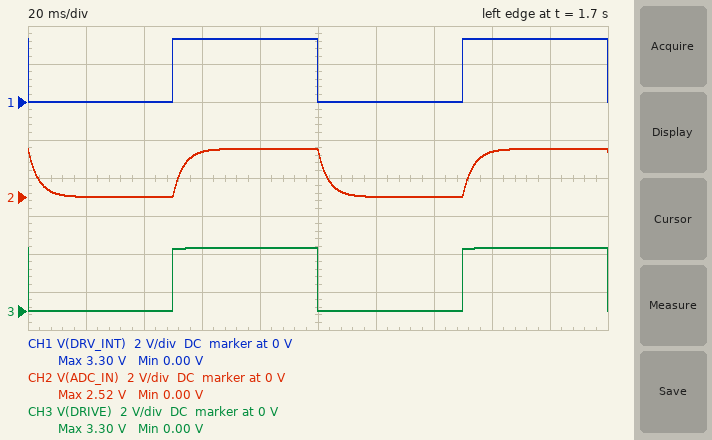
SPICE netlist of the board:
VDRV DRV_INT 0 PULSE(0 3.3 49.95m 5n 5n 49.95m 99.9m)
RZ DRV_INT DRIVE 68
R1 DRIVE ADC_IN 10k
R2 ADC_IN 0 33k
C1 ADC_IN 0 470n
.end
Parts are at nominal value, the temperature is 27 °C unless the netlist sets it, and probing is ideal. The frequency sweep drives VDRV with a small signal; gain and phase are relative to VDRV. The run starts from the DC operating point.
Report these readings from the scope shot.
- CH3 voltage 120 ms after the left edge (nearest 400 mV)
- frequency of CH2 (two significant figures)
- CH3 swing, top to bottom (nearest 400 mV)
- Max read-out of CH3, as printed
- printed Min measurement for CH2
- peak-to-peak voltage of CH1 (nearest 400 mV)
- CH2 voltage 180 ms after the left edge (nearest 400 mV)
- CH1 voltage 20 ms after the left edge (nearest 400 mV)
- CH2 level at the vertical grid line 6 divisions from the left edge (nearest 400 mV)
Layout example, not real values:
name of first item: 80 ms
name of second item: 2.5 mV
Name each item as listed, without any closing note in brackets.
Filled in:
CH3 voltage 120 ms after the left edge: 0 V
frequency of CH2: 10 Hz
CH3 swing, top to bottom: 3.2 V
Max read-out of CH3, as printed: 3.30 V
printed Min measurement for CH2: 0.00 V
peak-to-peak voltage of CH1: 3.2 V
CH2 voltage 180 ms after the left edge: 2.4 V
CH1 voltage 20 ms after the left edge: 0 V
CH2 level at the vertical grid line 6 divisions from the left edge: 0 V
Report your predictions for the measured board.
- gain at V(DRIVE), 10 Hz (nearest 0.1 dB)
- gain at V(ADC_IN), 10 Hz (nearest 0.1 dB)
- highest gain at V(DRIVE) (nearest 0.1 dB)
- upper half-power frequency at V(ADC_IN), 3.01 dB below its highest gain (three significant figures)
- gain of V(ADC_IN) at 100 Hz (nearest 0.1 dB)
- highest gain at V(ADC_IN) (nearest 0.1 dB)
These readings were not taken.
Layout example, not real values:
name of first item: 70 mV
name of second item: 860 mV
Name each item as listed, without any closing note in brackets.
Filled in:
gain at V(DRIVE), 10 Hz: 0 dB
gain at V(ADC_IN), 10 Hz: -2.5 dB
highest gain at V(DRIVE): 0 dB
upper half-power frequency at V(ADC_IN), 3.01 dB below its highest gain: 43.9 Hz
gain of V(ADC_IN) at 100 Hz: -10.2 dB
highest gain at V(ADC_IN): -2.3 dB
